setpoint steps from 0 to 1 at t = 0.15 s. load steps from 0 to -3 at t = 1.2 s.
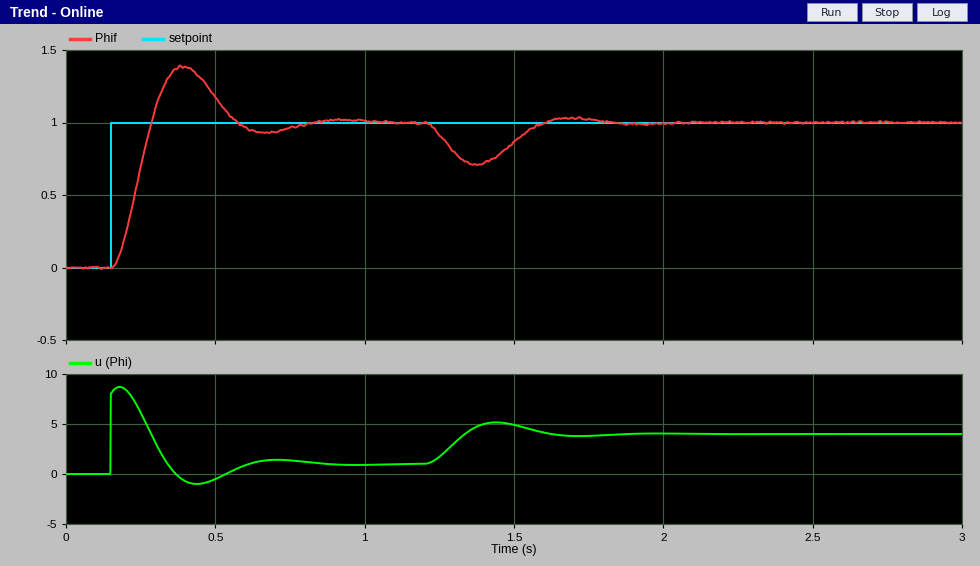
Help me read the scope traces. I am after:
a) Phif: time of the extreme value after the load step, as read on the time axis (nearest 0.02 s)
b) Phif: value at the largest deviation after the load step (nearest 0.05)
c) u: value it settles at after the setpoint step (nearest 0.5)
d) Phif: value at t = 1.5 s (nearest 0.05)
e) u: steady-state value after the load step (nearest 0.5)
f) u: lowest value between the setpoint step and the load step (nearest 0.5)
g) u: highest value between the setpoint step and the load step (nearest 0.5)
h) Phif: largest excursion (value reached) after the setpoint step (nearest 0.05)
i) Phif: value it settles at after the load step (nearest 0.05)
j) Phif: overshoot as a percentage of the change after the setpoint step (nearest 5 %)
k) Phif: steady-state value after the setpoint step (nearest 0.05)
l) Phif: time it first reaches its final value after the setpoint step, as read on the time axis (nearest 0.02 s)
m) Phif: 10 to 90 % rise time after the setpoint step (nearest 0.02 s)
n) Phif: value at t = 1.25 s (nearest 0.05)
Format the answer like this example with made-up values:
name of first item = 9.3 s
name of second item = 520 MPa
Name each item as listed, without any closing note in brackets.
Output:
Phif: time of the extreme value after the load step, as read on the time axis = 1.38 s
Phif: value at the largest deviation after the load step = 0.70
u: value it settles at after the setpoint step = 1.0
Phif: value at t = 1.5 s = 0.85
u: steady-state value after the load step = 4.0
u: lowest value between the setpoint step and the load step = -1.0
u: highest value between the setpoint step and the load step = 8.5
Phif: largest excursion (value reached) after the setpoint step = 1.40
Phif: value it settles at after the load step = 1.00
Phif: overshoot as a percentage of the change after the setpoint step = 40 %
Phif: steady-state value after the setpoint step = 1.00
Phif: time it first reaches its final value after the setpoint step, as read on the time axis = 0.28 s
Phif: 10 to 90 % rise time after the setpoint step = 0.10 s
Phif: value at t = 1.25 s = 0.90
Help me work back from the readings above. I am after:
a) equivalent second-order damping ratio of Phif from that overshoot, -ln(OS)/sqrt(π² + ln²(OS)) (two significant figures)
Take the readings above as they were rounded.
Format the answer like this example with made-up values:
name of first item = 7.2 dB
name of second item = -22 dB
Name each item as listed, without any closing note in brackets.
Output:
equivalent second-order damping ratio of Phif from that overshoot, -ln(OS)/sqrt(π² + ln²(OS)) = 0.28
